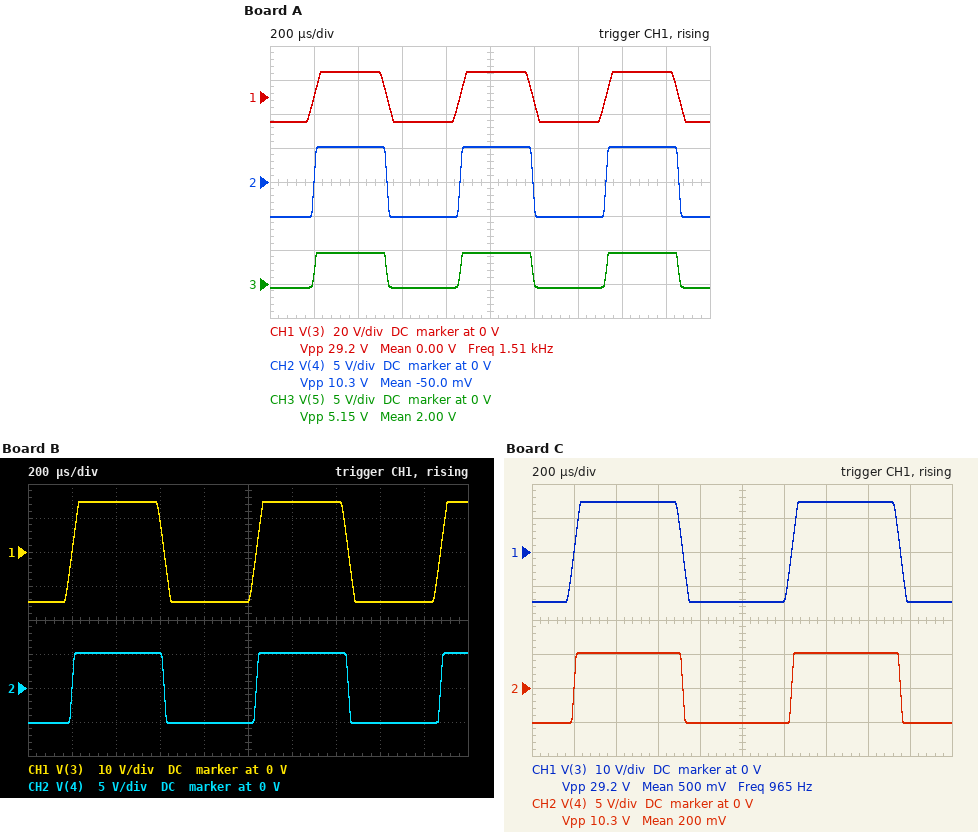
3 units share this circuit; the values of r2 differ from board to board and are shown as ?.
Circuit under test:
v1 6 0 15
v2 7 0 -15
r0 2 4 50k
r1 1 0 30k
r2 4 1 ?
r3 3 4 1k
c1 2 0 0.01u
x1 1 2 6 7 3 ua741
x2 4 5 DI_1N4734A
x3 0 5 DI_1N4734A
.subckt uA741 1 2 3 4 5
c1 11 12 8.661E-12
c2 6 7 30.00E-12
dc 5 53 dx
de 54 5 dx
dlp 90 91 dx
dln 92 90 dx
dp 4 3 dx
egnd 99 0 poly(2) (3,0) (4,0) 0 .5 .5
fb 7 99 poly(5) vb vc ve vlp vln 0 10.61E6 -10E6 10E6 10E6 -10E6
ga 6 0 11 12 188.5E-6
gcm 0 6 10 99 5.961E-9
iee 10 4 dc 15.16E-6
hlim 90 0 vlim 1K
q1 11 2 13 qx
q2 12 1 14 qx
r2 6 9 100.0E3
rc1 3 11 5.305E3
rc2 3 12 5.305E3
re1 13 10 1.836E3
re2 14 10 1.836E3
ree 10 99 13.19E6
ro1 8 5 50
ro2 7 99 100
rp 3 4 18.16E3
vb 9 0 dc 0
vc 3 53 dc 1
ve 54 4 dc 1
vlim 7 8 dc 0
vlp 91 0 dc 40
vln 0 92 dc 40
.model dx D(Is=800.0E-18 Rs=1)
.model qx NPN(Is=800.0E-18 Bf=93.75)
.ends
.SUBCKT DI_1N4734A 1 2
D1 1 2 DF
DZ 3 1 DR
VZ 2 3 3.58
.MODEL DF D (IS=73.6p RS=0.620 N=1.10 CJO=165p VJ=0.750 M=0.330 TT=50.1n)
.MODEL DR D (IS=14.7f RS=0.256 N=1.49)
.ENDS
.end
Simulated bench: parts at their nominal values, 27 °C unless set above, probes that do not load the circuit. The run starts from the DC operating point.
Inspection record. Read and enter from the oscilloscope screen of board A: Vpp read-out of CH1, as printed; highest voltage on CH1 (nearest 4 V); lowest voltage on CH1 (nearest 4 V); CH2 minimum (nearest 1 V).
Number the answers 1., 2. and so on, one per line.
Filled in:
1. 29.2 V
2. 16 V
3. -16 V
4. -5 V
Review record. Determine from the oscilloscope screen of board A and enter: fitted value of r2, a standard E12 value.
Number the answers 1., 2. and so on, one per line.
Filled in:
1. 82 kΩ
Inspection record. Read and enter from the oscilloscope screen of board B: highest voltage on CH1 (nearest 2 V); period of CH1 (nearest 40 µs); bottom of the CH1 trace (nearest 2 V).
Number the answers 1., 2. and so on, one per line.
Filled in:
1. 14 V
2. 840 µs
3. -14 V
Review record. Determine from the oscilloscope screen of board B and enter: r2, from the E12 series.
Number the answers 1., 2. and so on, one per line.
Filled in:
1. 56 kΩ
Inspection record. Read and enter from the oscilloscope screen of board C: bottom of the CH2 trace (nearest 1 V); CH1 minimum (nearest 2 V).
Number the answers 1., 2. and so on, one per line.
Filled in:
1. -5 V
2. -14 V
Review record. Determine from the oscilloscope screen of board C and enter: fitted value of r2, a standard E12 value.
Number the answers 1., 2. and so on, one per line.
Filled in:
1. 39 kΩ
